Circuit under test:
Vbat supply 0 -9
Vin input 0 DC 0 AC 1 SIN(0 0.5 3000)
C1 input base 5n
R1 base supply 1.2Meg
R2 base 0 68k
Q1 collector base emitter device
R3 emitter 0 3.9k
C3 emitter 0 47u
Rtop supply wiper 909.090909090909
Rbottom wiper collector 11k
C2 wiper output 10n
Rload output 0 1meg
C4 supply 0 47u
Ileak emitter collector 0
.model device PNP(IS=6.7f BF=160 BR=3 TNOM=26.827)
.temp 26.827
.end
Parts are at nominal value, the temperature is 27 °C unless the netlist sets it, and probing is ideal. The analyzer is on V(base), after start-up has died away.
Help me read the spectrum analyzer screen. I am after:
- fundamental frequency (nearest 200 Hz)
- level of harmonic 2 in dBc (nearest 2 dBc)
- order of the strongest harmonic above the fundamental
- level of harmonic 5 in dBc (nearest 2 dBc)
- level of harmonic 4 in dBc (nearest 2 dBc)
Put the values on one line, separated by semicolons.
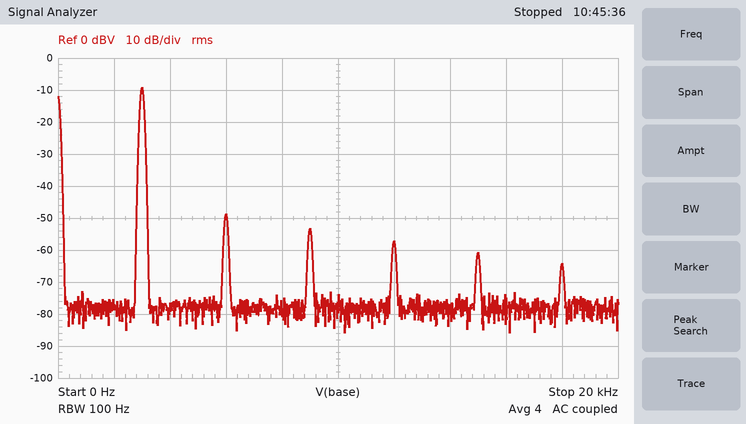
3.0 kHz; -40 dBc; 2; -52 dBc; -48 dBc
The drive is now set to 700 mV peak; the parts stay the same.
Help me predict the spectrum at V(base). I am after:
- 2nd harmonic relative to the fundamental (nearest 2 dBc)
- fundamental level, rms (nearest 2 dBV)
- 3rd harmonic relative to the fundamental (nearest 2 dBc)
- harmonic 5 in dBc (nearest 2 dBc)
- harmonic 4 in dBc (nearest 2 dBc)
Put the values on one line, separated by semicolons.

-32 dBc; -6 dBV; -36 dBc; -42 dBc; -40 dBc
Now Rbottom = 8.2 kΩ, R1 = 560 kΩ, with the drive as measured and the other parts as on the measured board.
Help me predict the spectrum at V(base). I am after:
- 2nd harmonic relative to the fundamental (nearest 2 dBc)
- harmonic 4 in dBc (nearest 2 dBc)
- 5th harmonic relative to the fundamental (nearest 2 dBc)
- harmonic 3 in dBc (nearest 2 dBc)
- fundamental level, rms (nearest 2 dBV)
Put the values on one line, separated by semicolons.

-26 dBc; -36 dBc; -40 dBc; -32 dBc; -10 dBV
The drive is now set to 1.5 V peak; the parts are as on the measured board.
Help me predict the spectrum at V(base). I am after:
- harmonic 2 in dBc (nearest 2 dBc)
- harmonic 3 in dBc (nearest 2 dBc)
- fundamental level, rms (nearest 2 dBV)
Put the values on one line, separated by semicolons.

-24 dBc; -28 dBc; 0 dBV
